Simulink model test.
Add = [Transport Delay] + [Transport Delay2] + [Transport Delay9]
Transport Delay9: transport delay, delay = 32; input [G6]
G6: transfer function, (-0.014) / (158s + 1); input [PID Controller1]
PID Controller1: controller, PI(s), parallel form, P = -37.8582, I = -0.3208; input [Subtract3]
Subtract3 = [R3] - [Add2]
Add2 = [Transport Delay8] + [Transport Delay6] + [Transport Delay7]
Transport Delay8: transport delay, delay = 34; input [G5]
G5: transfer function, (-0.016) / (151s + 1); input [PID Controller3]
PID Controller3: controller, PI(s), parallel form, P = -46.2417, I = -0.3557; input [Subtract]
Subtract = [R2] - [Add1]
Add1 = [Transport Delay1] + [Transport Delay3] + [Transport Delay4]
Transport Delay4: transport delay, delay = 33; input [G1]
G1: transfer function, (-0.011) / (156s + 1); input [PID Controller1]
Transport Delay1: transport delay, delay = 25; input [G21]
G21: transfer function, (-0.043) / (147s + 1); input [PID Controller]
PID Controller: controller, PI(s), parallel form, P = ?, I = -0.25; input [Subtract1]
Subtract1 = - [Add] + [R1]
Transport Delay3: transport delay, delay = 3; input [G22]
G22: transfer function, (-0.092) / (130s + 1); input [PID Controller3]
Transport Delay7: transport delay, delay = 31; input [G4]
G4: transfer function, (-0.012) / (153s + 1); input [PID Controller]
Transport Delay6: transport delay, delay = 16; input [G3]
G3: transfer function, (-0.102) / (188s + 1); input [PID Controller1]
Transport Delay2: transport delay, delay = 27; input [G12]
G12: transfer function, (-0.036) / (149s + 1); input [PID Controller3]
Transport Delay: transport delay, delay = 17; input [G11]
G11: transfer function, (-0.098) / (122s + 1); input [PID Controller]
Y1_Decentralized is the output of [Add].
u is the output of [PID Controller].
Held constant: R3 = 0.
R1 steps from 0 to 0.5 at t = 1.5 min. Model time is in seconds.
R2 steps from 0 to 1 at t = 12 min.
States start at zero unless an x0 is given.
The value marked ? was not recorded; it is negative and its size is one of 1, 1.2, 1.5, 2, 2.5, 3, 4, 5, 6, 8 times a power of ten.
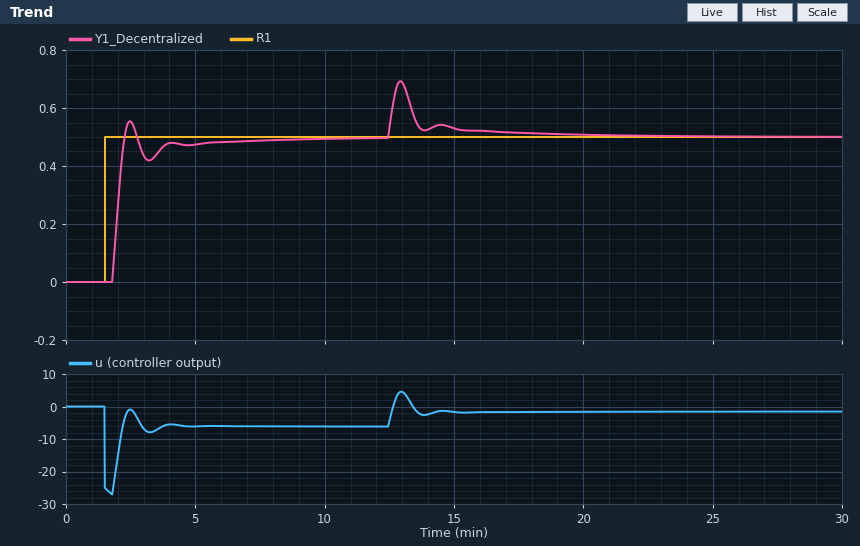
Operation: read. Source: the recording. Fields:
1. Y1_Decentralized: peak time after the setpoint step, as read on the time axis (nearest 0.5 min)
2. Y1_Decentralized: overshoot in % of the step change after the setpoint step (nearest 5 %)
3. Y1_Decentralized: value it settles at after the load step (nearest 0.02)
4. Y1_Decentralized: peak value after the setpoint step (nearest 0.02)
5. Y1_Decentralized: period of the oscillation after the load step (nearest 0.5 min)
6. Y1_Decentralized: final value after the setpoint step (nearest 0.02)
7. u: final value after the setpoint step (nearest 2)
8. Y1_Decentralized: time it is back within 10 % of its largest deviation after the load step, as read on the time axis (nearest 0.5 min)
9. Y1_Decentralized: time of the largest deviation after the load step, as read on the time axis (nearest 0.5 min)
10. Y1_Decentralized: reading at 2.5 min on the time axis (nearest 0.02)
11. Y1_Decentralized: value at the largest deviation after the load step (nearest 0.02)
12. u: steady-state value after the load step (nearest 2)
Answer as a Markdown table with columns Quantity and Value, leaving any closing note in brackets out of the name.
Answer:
| Quantity | Value |
|---|---|
| Y1_Decentralized: peak time after the setpoint step, as read on the time axis | 2.5 min |
| Y1_Decentralized: overshoot in % of the step change after the setpoint step | 10 % |
| Y1_Decentralized: value it settles at after the load step | 0.50 |
| Y1_Decentralized: peak value after the setpoint step | 0.56 |
| Y1_Decentralized: period of the oscillation after the load step | 1.5 min |
| Y1_Decentralized: final value after the setpoint step | 0.50 |
| u: final value after the setpoint step | -6 |
| Y1_Decentralized: time it is back within 10 % of its largest deviation after the load step, as read on the time axis | 16.5 min |
| Y1_Decentralized: time of the largest deviation after the load step, as read on the time axis | 13.0 min |
| Y1_Decentralized: reading at 2.5 min on the time axis | 0.56 |
| Y1_Decentralized: value at the largest deviation after the load step | 0.70 |
| u: steady-state value after the load step | -2 |
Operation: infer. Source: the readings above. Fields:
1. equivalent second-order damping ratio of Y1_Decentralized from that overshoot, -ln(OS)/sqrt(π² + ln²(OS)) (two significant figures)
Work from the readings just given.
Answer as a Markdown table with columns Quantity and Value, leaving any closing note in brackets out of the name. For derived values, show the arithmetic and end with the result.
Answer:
| Quantity | Value |
|---|---|
| equivalent second-order damping ratio of Y1_Decentralized from that overshoot, -ln(OS)/sqrt(π² + ln²(OS)) | ln(0.1) = -2.303; 2.303 / sqrt(9.870 + 5.302) = 0.59 |
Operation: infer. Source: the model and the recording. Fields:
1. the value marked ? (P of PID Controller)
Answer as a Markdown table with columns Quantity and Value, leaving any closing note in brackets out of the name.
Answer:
| Quantity | Value |
|---|---|
| the value marked ? | -50 |
